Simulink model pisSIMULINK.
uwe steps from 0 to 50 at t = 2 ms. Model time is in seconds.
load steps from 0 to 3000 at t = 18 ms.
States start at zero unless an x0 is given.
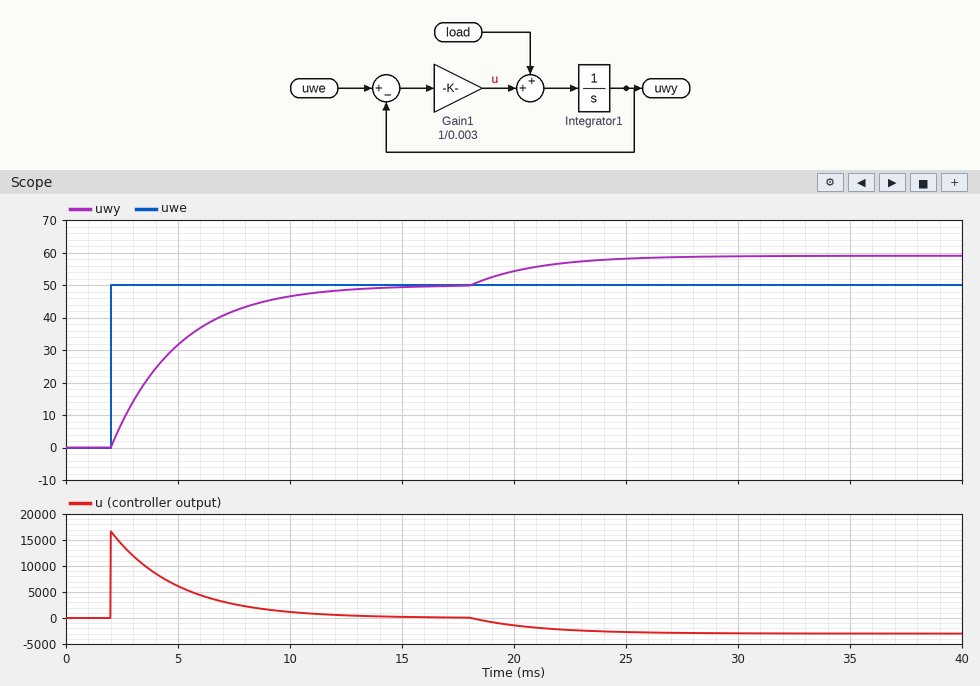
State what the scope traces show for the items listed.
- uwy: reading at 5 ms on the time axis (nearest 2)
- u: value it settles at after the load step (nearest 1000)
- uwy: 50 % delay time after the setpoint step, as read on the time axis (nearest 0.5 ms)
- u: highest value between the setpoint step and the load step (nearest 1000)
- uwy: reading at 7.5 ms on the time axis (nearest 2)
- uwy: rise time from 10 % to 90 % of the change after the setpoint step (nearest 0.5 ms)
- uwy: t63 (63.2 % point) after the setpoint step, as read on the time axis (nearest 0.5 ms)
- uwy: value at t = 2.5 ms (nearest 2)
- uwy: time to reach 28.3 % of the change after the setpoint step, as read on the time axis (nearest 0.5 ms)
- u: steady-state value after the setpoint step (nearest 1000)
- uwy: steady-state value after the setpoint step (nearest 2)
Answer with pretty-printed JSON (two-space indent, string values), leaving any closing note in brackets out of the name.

{
  "uwy: reading at 5 ms on the time axis": "32",
  "u: value it settles at after the load step": "-3000",
  "uwy: 50 % delay time after the setpoint step, as read on the time axis": "4.0 ms",
  "u: highest value between the setpoint step and the load step": "17000",
  "uwy: reading at 7.5 ms on the time axis": "42",
  "uwy: rise time from 10 % to 90 % of the change after the setpoint step": "6.5 ms",
  "uwy: t63 (63.2 % point) after the setpoint step, as read on the time axis": "5.0 ms",
  "uwy: value at t = 2.5 ms": "8",
  "uwy: time to reach 28.3 % of the change after the setpoint step, as read on the time axis": "3.0 ms",
  "u: steady-state value after the setpoint step": "0",
  "uwy: steady-state value after the setpoint step": "50"
}
